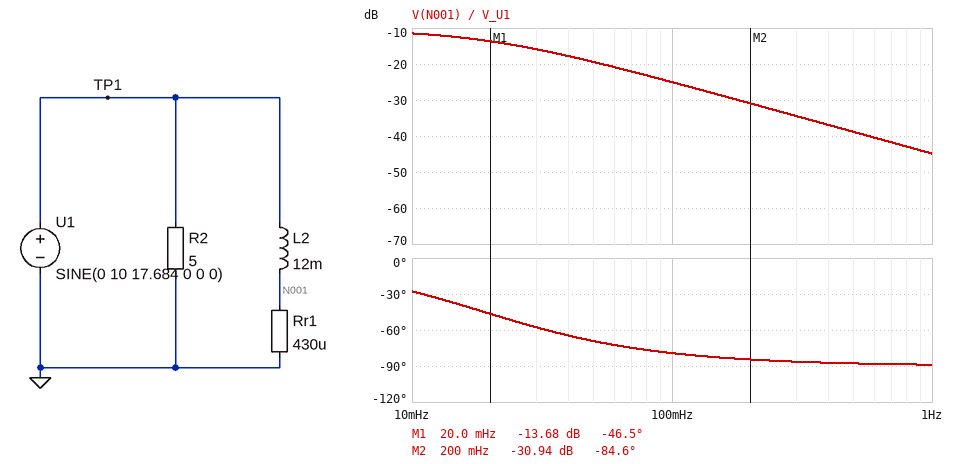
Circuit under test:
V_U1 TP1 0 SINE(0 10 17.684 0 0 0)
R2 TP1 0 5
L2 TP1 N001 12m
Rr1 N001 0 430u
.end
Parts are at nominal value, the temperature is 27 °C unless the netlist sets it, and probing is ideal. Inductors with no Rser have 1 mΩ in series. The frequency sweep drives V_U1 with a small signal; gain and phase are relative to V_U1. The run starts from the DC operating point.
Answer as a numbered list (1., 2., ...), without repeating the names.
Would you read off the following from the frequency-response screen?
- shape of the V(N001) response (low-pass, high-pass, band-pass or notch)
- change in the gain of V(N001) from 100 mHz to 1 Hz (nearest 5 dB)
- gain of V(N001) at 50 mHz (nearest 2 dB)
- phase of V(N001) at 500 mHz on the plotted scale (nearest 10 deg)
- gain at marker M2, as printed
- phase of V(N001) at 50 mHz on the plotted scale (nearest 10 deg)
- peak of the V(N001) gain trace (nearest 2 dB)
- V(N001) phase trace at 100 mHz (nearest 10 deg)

1. low-pass
2. -20 dB
3. -20 dB
4. -90 deg
5. -30.94 dB
6. -70 deg
7. -12 dB
8. -80 deg
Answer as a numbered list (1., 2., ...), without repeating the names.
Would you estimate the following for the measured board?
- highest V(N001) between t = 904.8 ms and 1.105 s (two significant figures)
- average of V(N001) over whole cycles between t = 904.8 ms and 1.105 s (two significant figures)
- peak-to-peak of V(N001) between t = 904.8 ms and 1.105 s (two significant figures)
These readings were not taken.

1. 6.1 mV
2. 2.9 mV
3. 6.5 mV
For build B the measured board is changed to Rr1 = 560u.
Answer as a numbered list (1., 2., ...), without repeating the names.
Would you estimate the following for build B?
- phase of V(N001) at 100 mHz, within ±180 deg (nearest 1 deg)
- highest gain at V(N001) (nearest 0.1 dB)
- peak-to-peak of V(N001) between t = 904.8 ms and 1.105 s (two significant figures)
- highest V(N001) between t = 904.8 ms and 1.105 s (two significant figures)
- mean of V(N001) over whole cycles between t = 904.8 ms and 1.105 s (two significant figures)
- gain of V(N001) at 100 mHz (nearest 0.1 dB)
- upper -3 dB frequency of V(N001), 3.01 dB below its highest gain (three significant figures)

1. -78 deg
2. -8.9 dB
3. 8.5 mV
4. 7.9 mV
5. 3.7 mV
6. -22.8 dB
7. 20.7 mHz
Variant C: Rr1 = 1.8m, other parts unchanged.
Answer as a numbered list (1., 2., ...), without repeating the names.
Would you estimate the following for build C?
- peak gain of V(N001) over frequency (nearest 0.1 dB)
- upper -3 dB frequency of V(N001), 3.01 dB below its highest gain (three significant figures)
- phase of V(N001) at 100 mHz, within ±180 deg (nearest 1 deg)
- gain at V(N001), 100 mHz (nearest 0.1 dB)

1. -3.8 dB
2. 37.1 mHz
3. -70 deg
4. -13.0 dB
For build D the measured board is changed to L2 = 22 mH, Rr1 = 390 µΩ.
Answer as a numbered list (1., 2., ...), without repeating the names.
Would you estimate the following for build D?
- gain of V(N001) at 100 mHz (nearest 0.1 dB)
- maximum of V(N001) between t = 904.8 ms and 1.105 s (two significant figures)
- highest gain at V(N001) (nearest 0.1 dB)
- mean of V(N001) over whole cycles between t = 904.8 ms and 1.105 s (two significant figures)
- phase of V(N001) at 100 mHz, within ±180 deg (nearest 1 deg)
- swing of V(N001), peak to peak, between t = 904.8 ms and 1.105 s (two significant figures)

1. -31.0 dB
2. 3.1 mV
3. -11.0 dB
4. 1.5 mV
5. -84 deg
6. 3.2 mV
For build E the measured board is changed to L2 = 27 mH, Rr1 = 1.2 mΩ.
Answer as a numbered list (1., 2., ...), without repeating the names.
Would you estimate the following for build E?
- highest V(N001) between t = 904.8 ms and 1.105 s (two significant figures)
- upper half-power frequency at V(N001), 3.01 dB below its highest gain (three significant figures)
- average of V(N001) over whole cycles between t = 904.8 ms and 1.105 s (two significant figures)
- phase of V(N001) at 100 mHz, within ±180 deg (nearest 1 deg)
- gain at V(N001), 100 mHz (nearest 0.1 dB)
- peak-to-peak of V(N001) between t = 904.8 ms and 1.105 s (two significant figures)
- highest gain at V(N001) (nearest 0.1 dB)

1. 7.7 mV
2. 13.0 mHz
3. 3.7 mV
4. -83 deg
5. -23.1 dB
6. 8.0 mV
7. -5.3 dB
